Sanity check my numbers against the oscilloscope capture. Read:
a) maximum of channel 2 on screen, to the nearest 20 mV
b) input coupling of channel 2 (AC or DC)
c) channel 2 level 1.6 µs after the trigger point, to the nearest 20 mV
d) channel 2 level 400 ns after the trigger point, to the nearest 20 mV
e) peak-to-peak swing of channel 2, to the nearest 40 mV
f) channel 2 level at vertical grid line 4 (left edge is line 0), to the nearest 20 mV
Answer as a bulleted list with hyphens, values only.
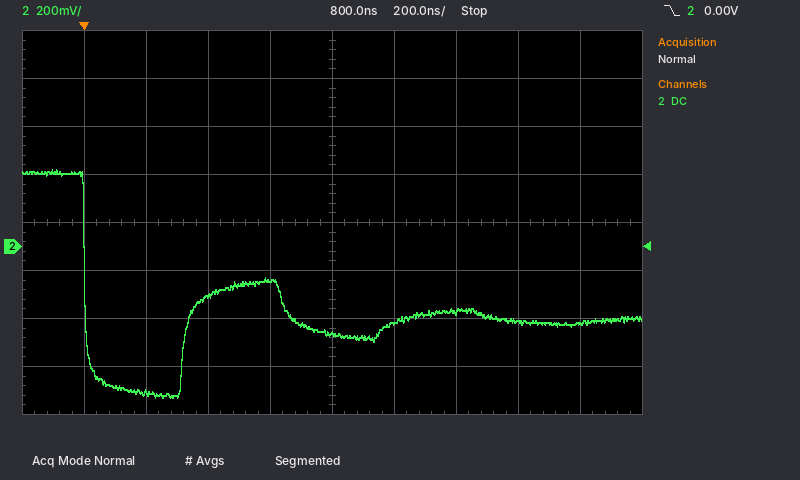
- 320 mV
- DC
- -320 mV
- -200 mV
- 960 mV
- -140 mV
